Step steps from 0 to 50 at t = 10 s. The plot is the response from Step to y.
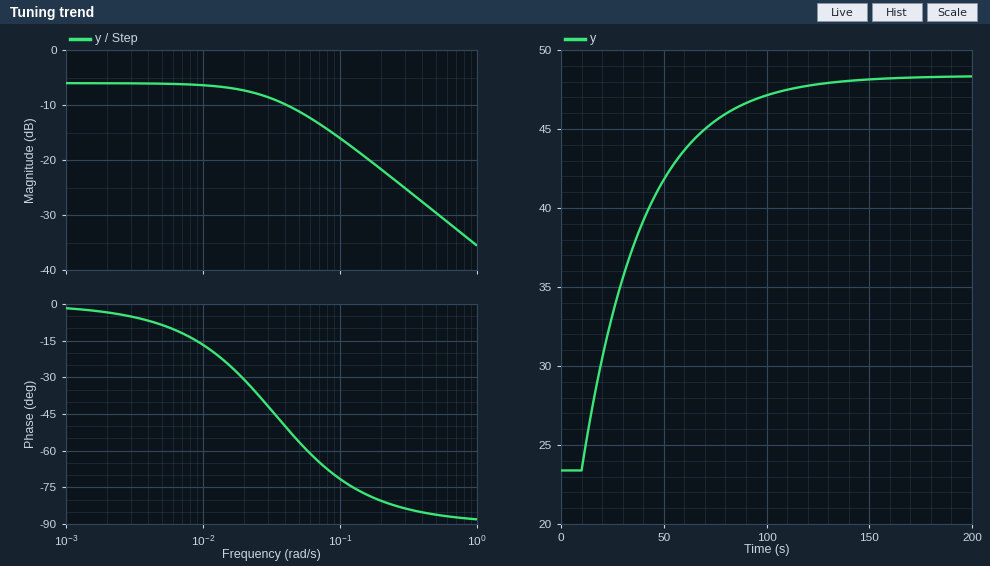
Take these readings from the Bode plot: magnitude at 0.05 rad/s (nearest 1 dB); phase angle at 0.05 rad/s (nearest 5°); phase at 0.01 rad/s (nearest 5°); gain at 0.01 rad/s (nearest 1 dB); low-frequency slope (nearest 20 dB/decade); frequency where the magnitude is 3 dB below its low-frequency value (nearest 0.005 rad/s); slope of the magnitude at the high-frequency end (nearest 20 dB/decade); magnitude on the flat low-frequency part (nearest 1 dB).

-11 dB
-55°
-15°
-6 dB
0 dB/decade
0.035 rad/s
-20 dB/decade
-6 dB
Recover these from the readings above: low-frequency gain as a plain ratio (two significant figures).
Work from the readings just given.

0.50
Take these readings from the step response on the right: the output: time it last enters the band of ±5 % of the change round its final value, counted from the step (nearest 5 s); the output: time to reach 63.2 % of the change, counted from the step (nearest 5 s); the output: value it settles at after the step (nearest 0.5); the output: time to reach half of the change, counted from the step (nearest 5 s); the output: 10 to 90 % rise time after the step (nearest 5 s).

90 s
30 s
48.5
20 s
65 s
